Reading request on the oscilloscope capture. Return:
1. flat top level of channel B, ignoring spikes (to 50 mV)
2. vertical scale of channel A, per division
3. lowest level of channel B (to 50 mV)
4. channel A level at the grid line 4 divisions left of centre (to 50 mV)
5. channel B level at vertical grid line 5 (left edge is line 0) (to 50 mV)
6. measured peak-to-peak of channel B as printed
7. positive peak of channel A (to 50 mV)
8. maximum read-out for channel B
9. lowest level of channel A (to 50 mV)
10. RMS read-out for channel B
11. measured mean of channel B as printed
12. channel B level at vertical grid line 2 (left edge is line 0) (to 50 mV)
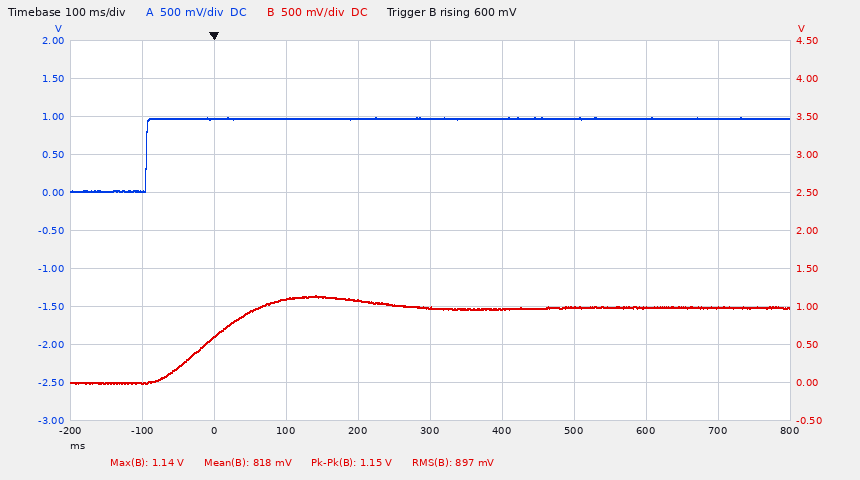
1.00 V
500 mV
0 mV
0 mV
1.00 V
1.15 V
1.00 V
1.14 V
0 mV
897 mV
818 mV
600 mV
